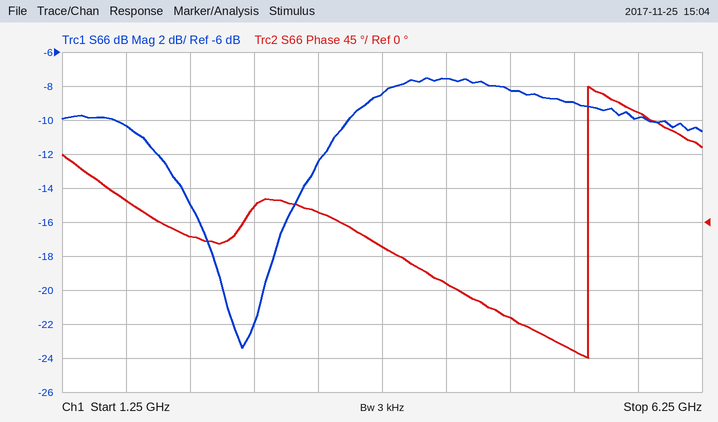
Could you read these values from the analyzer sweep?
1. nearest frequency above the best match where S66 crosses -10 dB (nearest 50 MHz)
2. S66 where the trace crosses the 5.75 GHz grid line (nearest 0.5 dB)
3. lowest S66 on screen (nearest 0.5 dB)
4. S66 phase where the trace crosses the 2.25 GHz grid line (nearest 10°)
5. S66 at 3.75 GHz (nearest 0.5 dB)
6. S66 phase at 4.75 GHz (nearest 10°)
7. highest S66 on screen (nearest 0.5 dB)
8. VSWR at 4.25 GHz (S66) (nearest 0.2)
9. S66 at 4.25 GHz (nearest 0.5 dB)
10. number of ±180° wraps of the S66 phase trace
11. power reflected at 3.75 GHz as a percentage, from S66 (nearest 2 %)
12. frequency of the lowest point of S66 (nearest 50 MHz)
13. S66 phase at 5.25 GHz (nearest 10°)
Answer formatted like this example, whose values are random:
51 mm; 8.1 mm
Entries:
3.50 GHz; -10.0 dB; -23.5 dB; -20°; -8.5 dB; -130°; -7.5 dB; 2.4; -7.5 dB; 1; 14 %; 2.65 GHz; -170°
